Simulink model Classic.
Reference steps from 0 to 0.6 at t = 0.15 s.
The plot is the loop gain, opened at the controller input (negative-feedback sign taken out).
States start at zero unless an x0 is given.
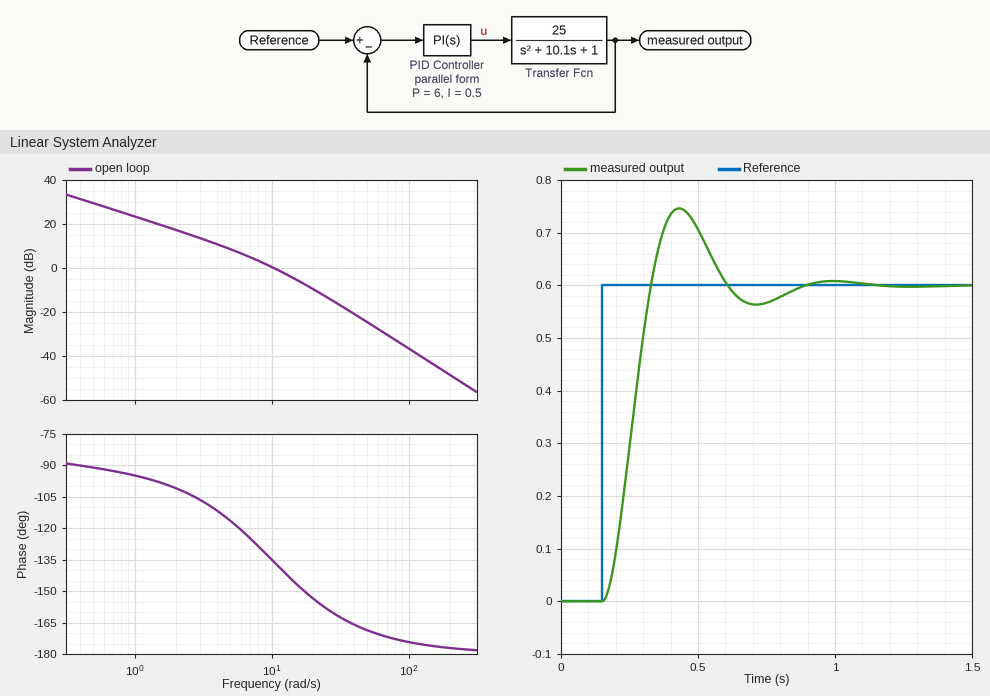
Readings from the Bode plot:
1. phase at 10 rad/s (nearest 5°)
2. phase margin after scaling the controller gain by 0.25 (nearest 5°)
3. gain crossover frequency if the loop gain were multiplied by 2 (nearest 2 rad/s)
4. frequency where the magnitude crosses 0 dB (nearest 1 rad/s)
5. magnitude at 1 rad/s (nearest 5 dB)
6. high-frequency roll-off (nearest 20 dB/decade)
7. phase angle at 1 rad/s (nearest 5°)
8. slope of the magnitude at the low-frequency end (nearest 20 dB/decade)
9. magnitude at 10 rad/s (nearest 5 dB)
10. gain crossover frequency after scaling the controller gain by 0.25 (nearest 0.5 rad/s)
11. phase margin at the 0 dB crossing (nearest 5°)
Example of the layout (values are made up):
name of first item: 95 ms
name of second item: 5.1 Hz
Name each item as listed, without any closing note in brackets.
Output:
phase at 10 rad/s: -135°
phase margin after scaling the controller gain by 0.25: 70°
gain crossover frequency if the loop gain were multiplied by 2: 16 rad/s
frequency where the magnitude crosses 0 dB: 10 rad/s
magnitude at 1 rad/s: 25 dB
high-frequency roll-off: -40 dB/decade
phase angle at 1 rad/s: -95°
slope of the magnitude at the low-frequency end: -20 dB/decade
magnitude at 10 rad/s: 0 dB
gain crossover frequency after scaling the controller gain by 0.25: 3.5 rad/s
phase margin at the 0 dB crossing: 45°
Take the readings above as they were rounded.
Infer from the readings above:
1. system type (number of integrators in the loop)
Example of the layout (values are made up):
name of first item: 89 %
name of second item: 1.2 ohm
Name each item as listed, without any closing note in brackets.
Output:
system type: 1
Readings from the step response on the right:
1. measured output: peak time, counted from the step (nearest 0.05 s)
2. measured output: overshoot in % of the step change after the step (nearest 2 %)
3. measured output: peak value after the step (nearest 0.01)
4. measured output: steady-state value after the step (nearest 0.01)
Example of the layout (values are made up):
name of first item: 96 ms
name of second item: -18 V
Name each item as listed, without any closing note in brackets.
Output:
measured output: peak time, counted from the step: 0.30 s
measured output: overshoot in % of the step change after the step: 24 %
measured output: peak value after the step: 0.75
measured output: steady-state value after the step: 0.60
